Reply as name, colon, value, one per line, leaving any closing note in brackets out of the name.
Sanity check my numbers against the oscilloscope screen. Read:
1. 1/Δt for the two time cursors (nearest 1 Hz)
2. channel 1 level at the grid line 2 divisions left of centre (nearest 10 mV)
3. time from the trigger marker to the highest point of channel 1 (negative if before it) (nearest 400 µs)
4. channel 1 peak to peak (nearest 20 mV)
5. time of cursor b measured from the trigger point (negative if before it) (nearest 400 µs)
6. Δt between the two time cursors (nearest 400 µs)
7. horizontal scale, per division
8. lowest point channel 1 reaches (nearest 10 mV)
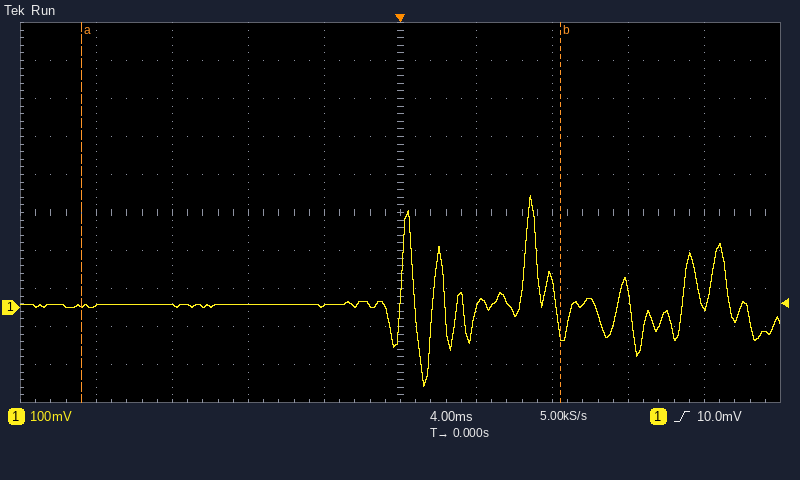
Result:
1/Δt for the two time cursors: 40 Hz
channel 1 level at the grid line 2 divisions left of centre: 10 mV
time from the trigger marker to the highest point of channel 1 (negative if before it): +6.8 ms
channel 1 peak to peak: 500 mV
time of cursor b measured from the trigger point (negative if before it): +8.4 ms
Δt between the two time cursors: 25.2 ms
horizontal scale, per division: 4 ms
lowest point channel 1 reaches: -210 mV
